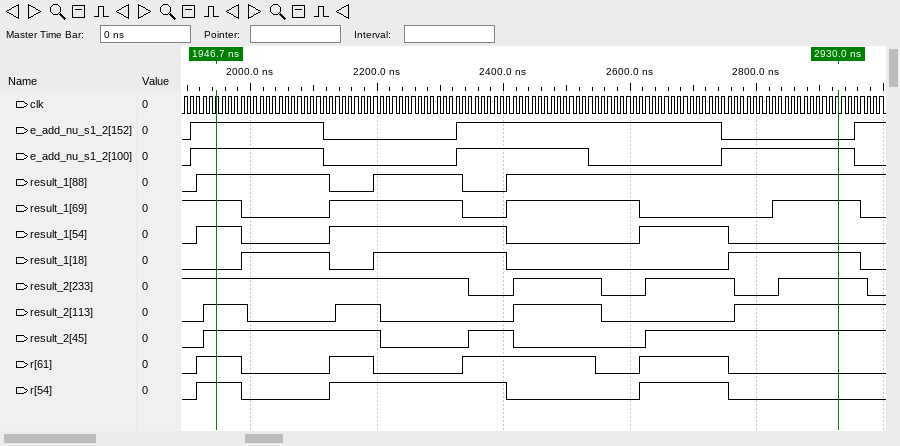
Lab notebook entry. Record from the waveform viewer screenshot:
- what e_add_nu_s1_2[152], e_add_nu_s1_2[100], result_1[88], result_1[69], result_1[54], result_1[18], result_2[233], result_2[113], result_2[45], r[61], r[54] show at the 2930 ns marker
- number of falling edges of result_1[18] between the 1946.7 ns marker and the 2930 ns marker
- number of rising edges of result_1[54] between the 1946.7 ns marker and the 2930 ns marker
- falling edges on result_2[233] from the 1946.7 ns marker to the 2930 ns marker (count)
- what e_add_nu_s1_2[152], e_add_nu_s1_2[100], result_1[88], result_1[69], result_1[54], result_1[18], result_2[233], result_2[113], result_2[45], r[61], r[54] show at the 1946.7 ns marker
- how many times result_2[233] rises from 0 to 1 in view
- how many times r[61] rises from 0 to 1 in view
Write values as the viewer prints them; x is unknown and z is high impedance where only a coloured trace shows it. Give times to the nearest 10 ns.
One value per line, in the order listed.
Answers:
e_add_nu_s1_2[152]=0, e_add_nu_s1_2[100]=1, result_1[88]=1, result_1[69]=1, result_1[54]=0, result_1[18]=1, result_2[233]=1, result_2[113]=1, result_2[45]=1, r[61]=0, r[54]=0
2
2
3
e_add_nu_s1_2[152]=1, e_add_nu_s1_2[100]=1, result_1[88]=1, result_1[69]=1, result_1[54]=1, result_1[18]=0, result_2[233]=1, result_2[113]=1, result_2[45]=1, r[61]=1, r[54]=1
3
4
